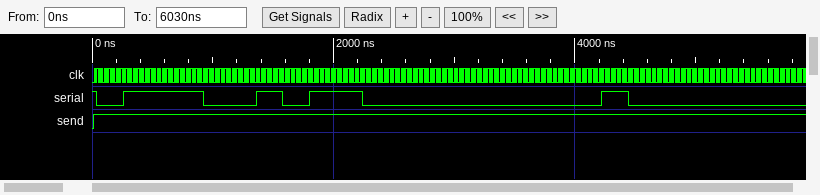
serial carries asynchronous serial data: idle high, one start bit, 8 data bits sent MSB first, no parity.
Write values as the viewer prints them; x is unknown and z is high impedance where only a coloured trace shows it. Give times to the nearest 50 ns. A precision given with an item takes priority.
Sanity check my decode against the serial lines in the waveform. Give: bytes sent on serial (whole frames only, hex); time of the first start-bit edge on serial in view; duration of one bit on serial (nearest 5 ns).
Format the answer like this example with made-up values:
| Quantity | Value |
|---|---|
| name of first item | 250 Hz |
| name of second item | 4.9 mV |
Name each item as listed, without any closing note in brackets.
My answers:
| Quantity | Value |
|---|---|
| bytes sent on serial | E5, 00 |
| time of the first start-bit edge on serial in view | 0 ns |
| duration of one bit on serial | 220 ns |
